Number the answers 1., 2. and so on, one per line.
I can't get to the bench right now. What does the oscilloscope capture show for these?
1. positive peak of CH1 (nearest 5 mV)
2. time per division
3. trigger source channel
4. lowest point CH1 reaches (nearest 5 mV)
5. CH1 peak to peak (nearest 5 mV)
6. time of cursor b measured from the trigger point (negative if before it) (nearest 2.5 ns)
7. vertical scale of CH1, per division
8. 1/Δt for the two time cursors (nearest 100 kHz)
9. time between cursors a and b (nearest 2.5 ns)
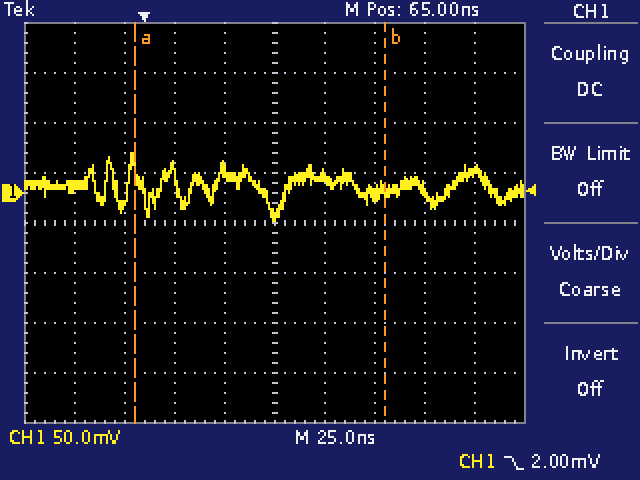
1. 40 mV
2. 25 ns
3. CH1
4. -30 mV
5. 70 mV
6. +120.0 ns
7. 50 mV
8. 8.0 MHz
9. 125.0 ns
